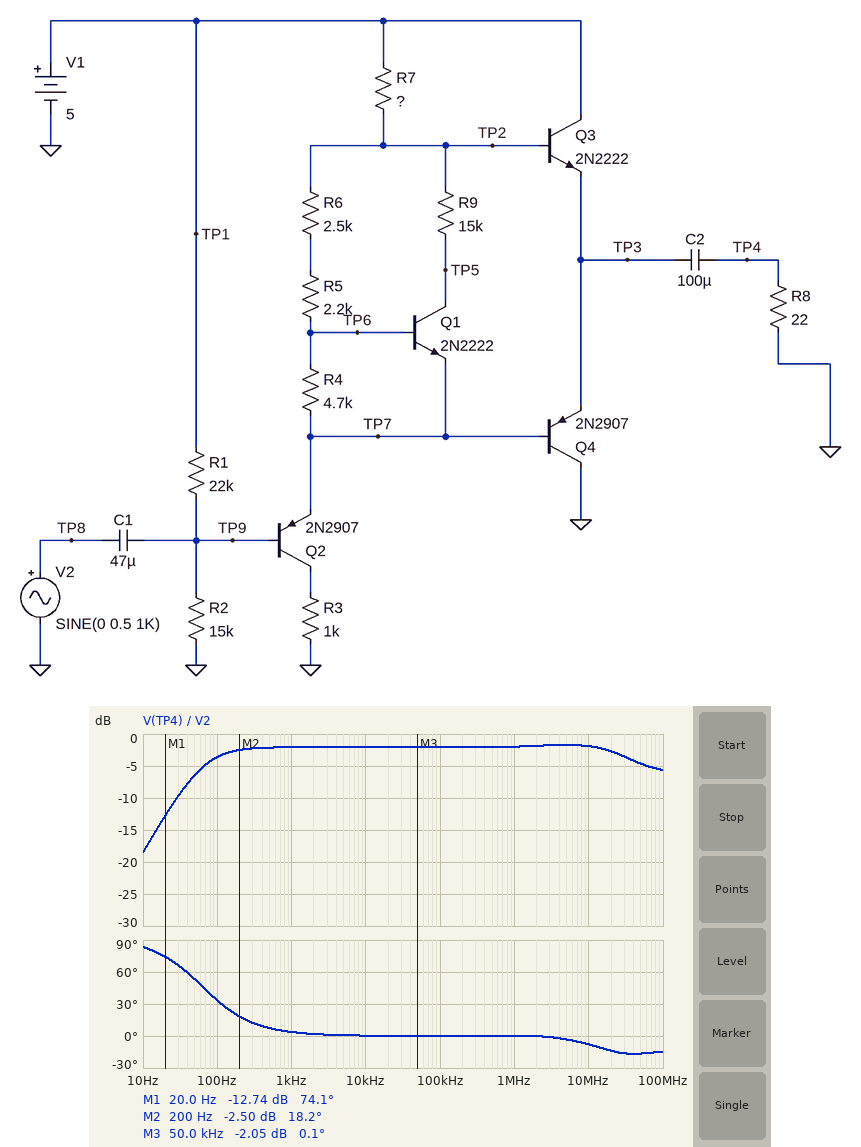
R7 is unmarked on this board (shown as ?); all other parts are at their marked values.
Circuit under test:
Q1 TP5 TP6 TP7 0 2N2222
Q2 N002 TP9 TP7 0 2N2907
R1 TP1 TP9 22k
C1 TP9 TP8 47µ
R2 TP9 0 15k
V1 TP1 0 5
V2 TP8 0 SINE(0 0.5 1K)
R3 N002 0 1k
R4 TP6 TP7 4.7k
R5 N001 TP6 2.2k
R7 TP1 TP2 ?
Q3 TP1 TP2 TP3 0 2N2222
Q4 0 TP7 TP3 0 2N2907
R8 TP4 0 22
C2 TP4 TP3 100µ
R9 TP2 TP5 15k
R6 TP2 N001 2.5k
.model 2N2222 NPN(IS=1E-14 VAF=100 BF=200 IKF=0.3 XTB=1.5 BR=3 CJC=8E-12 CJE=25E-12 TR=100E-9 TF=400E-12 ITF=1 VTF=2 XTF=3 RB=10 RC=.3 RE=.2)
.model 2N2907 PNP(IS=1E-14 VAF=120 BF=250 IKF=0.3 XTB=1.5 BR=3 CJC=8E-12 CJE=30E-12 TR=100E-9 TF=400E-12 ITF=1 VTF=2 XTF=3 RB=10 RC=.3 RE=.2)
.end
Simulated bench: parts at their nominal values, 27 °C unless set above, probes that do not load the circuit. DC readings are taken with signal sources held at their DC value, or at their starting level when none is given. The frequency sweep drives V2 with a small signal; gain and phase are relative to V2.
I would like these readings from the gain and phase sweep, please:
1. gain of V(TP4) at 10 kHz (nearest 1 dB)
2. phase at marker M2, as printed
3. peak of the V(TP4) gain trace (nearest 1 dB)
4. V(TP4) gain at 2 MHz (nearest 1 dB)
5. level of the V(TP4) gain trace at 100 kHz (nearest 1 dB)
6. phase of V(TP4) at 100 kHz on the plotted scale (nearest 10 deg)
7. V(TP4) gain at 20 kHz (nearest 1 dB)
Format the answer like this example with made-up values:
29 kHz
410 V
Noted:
-2 dB
18.2 deg
-2 dB
-2 dB
-2 dB
0 deg
-2 dB
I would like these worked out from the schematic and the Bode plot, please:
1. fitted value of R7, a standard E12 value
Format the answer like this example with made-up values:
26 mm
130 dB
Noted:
2.7 kΩ
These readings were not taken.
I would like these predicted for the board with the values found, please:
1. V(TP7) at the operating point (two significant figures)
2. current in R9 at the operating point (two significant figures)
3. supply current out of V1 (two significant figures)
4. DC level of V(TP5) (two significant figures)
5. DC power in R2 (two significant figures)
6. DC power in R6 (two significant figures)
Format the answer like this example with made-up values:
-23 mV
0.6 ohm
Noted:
2.7 V
95 µA
12 mA
2.7 V
280 µW
77 µW
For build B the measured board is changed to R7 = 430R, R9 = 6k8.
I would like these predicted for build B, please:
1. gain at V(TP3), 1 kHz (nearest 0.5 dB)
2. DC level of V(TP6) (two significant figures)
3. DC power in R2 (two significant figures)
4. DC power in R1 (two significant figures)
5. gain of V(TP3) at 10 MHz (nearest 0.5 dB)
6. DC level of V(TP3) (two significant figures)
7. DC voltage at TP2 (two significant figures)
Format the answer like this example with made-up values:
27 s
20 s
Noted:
-1.5 dB
3.4 V
290 µW
390 µW
-1.0 dB
3.6 V
4.4 V
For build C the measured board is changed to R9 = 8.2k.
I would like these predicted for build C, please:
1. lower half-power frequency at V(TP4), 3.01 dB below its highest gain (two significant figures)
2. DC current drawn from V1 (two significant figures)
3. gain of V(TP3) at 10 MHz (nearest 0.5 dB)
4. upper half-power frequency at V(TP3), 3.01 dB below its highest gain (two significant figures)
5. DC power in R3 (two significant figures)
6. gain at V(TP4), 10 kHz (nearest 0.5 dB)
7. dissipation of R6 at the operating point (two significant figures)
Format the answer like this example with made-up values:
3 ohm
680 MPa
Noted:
65 Hz
4.8 mA
-3.0 dB
29 MHz
120 µW
-3.5 dB
66 µW
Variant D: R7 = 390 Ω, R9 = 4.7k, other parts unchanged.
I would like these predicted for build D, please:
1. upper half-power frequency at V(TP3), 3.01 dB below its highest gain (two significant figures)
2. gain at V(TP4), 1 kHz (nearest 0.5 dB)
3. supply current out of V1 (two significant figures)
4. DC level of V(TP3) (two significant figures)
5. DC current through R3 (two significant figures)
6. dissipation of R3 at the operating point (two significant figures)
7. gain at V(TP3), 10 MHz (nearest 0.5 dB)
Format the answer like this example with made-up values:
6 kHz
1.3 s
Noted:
110 MHz
-1.5 dB
140 mA
3.6 V
1.3 mA
1.8 mW
-1.0 dB
